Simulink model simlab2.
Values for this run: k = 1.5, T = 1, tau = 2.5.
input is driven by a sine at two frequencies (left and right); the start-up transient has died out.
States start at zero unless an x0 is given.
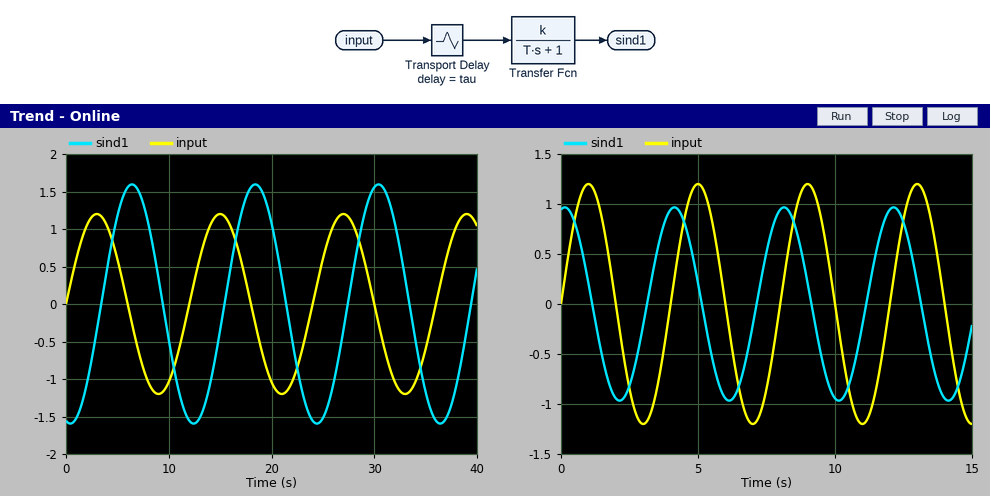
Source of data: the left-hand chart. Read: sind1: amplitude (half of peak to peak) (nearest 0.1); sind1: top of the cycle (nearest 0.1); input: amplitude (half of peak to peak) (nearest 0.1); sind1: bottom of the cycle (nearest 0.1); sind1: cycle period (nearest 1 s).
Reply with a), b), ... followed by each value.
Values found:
a) 1.6
b) 1.6
c) 1.2
d) -1.6
e) 12 s
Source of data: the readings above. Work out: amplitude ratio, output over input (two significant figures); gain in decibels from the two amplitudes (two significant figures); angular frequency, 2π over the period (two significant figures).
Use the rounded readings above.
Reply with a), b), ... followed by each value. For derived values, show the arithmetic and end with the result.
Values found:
a) 1.6 / 1.2 = 1.3
b) 20 log10(1.6 / 1.2) = 2.5 dB
c) 2π / 12 = 0.52 rad/s
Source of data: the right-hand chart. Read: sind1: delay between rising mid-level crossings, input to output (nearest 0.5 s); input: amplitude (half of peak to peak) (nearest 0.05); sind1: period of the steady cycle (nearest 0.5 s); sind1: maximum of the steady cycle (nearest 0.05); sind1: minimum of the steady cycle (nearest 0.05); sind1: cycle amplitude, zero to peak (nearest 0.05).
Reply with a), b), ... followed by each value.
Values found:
a) 3.0 s
b) 1.20
c) 4.0 s
d) 0.95
e) -0.95
f) 0.95
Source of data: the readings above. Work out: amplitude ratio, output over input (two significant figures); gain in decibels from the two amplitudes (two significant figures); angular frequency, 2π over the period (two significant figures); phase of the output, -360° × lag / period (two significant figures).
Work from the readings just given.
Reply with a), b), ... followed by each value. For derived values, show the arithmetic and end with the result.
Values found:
a) 0.95 / 1.2 = 0.79
b) 20 log10(0.95 / 1.2) = -2.0 dB
c) 2π / 4 = 1.6 rad/s
d) -360 × 3 / 4 = -270°
